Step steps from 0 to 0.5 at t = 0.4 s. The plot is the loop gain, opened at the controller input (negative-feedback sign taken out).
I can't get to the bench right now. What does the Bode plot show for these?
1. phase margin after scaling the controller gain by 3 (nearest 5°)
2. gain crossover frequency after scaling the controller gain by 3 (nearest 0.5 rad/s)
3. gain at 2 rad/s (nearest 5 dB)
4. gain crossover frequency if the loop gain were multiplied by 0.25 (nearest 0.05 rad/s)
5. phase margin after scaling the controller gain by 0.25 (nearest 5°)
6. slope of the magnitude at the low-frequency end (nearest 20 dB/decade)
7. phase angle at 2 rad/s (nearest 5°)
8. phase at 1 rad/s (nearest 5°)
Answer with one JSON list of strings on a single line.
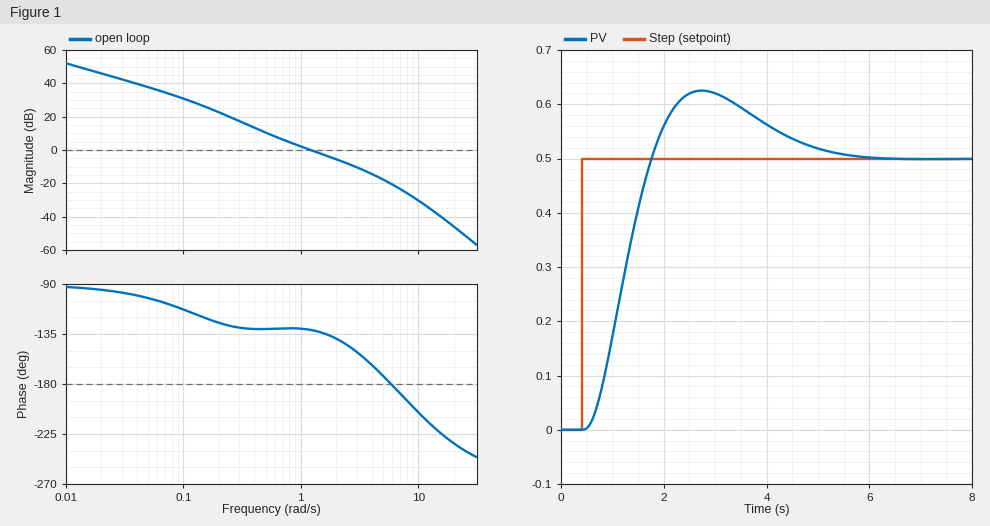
["30°", "3.0 rad/s", "-5 dB", "0.45 rad/s", "50°", "-20 dB/decade", "-140°", "-130°"]
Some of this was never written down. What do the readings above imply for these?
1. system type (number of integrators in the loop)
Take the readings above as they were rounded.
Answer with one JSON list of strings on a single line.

["1"]
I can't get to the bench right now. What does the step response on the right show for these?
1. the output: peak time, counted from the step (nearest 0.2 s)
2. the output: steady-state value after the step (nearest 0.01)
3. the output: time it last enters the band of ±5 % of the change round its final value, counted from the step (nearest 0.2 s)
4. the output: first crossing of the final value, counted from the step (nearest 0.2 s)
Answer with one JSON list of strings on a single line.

["2.4 s", "0.50", "4.4 s", "1.4 s"]
